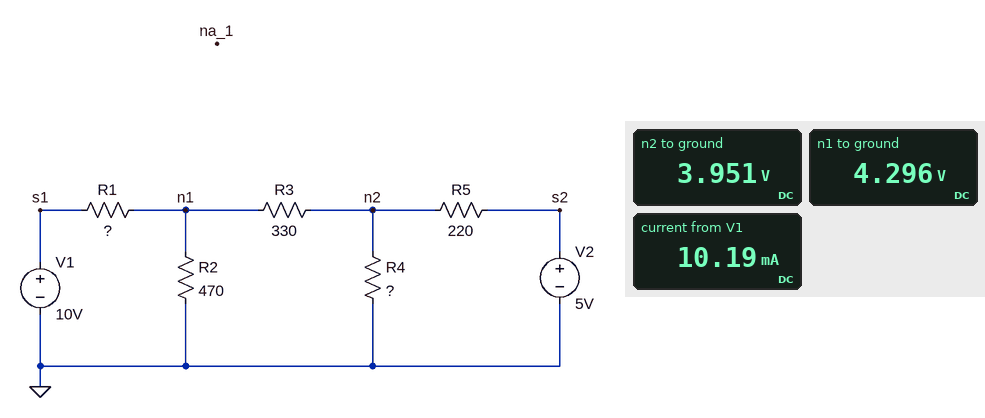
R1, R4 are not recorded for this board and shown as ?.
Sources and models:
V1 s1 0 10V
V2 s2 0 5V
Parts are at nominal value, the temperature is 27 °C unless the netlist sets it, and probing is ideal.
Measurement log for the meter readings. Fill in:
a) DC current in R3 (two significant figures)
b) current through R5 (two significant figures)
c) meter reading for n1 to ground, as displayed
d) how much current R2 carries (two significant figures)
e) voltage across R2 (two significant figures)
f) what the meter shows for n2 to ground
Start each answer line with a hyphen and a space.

- 1.0 mA
- 4.8 mA
- 4.296 V
- 9.1 mA
- 4.3 V
- 3.951 V
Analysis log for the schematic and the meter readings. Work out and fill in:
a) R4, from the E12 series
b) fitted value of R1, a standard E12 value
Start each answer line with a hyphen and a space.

- 680 Ω
- 560 Ω
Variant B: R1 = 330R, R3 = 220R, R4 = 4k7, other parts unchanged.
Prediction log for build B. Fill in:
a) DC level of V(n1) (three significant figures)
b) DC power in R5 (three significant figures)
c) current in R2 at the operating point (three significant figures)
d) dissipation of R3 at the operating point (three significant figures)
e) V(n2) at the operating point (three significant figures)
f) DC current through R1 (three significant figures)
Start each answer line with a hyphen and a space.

- 5.53 V
- 97.4 µW
- 11.8 mA
- 682 µW
- 5.15 V
- 13.5 mA
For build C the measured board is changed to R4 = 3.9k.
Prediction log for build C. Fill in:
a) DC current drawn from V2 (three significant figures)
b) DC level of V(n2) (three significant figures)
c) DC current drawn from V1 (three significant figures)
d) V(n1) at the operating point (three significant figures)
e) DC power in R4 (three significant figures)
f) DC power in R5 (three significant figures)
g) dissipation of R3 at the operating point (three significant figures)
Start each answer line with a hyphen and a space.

- 1.42 mA
- 4.69 V
- 9.61 mA
- 4.62 V
- 5.64 mW
- 441 µW
- 15.1 µW
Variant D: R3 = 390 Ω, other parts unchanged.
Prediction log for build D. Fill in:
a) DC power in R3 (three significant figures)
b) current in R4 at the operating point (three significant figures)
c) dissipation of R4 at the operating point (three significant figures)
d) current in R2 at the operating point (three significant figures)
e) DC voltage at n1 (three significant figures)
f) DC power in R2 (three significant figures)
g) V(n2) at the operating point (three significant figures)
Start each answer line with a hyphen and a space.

- 365 µW
- 5.79 mA
- 22.8 mW
- 9.18 mA
- 4.32 V
- 39.6 mW
- 3.94 V
